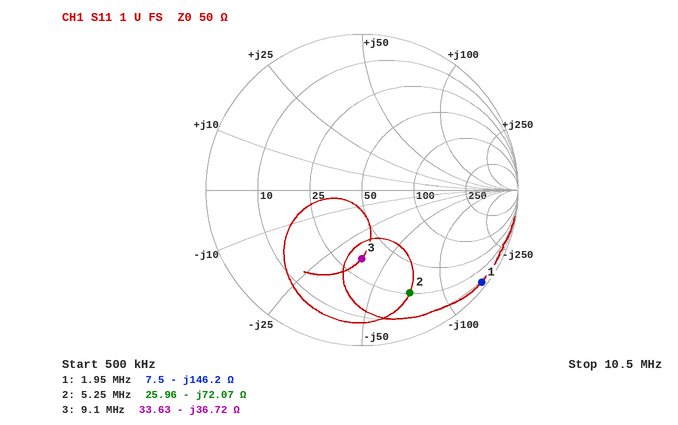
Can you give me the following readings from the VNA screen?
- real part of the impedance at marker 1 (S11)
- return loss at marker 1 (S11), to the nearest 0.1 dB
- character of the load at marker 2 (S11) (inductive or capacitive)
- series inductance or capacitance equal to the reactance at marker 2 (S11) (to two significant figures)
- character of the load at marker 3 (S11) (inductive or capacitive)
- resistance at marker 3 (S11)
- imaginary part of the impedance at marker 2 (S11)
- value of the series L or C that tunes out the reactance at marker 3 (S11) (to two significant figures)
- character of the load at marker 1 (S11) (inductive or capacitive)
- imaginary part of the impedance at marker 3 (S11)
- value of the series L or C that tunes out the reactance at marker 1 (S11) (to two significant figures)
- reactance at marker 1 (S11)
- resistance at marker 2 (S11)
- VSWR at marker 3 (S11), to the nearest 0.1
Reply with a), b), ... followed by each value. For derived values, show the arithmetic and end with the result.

a) 7.5 Ω
b) 0.3 dB
c) capacitive
d) C = 1/(2π × 5.25 MHz × 72.07 Ω) ≈ 421 pF, so 420 pF to two significant figures
e) capacitive
f) 33.63 Ω
g) -72.07 Ω
h) L = 36.72 Ω/(2π × 9.1 MHz) ≈ 642 nH, so 640 nH to two significant figures
i) capacitive
j) -36.72 Ω
k) L = 146.2 Ω/(2π × 1.95 MHz) ≈ 12 µH
l) -146.2 Ω
m) 25.96 Ω
n) 2.6
